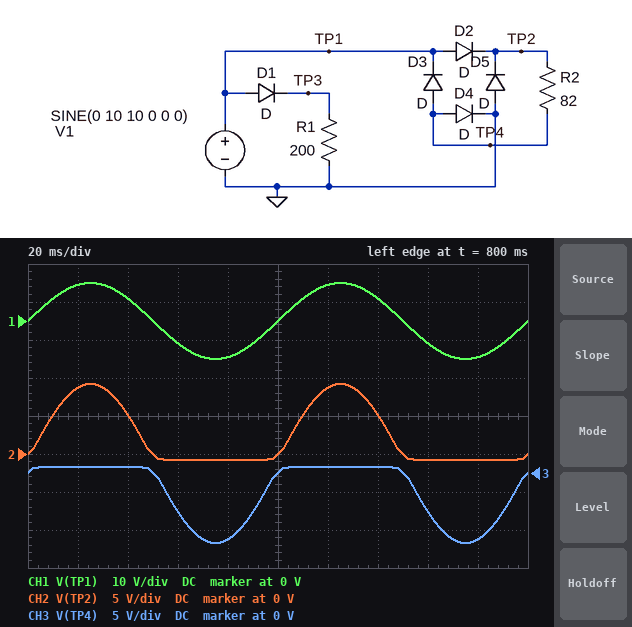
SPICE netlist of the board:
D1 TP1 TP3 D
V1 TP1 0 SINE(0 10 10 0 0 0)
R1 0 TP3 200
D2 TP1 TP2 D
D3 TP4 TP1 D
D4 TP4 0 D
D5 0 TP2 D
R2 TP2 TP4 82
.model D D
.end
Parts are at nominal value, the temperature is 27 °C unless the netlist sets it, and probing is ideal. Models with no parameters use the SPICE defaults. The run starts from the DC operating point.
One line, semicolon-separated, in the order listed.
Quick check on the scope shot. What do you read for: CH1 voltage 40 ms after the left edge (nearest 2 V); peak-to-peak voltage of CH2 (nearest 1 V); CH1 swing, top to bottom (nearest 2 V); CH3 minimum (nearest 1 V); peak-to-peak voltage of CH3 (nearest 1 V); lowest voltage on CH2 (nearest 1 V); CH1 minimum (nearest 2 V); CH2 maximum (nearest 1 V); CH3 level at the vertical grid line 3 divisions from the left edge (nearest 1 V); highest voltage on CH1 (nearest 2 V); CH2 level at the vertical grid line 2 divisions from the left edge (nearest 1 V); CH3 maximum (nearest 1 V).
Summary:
6 V; 10 V; 20 V; -9 V; 10 V; -1 V; -10 V; 9 V; -5 V; 10 V; 5 V; 1 V
